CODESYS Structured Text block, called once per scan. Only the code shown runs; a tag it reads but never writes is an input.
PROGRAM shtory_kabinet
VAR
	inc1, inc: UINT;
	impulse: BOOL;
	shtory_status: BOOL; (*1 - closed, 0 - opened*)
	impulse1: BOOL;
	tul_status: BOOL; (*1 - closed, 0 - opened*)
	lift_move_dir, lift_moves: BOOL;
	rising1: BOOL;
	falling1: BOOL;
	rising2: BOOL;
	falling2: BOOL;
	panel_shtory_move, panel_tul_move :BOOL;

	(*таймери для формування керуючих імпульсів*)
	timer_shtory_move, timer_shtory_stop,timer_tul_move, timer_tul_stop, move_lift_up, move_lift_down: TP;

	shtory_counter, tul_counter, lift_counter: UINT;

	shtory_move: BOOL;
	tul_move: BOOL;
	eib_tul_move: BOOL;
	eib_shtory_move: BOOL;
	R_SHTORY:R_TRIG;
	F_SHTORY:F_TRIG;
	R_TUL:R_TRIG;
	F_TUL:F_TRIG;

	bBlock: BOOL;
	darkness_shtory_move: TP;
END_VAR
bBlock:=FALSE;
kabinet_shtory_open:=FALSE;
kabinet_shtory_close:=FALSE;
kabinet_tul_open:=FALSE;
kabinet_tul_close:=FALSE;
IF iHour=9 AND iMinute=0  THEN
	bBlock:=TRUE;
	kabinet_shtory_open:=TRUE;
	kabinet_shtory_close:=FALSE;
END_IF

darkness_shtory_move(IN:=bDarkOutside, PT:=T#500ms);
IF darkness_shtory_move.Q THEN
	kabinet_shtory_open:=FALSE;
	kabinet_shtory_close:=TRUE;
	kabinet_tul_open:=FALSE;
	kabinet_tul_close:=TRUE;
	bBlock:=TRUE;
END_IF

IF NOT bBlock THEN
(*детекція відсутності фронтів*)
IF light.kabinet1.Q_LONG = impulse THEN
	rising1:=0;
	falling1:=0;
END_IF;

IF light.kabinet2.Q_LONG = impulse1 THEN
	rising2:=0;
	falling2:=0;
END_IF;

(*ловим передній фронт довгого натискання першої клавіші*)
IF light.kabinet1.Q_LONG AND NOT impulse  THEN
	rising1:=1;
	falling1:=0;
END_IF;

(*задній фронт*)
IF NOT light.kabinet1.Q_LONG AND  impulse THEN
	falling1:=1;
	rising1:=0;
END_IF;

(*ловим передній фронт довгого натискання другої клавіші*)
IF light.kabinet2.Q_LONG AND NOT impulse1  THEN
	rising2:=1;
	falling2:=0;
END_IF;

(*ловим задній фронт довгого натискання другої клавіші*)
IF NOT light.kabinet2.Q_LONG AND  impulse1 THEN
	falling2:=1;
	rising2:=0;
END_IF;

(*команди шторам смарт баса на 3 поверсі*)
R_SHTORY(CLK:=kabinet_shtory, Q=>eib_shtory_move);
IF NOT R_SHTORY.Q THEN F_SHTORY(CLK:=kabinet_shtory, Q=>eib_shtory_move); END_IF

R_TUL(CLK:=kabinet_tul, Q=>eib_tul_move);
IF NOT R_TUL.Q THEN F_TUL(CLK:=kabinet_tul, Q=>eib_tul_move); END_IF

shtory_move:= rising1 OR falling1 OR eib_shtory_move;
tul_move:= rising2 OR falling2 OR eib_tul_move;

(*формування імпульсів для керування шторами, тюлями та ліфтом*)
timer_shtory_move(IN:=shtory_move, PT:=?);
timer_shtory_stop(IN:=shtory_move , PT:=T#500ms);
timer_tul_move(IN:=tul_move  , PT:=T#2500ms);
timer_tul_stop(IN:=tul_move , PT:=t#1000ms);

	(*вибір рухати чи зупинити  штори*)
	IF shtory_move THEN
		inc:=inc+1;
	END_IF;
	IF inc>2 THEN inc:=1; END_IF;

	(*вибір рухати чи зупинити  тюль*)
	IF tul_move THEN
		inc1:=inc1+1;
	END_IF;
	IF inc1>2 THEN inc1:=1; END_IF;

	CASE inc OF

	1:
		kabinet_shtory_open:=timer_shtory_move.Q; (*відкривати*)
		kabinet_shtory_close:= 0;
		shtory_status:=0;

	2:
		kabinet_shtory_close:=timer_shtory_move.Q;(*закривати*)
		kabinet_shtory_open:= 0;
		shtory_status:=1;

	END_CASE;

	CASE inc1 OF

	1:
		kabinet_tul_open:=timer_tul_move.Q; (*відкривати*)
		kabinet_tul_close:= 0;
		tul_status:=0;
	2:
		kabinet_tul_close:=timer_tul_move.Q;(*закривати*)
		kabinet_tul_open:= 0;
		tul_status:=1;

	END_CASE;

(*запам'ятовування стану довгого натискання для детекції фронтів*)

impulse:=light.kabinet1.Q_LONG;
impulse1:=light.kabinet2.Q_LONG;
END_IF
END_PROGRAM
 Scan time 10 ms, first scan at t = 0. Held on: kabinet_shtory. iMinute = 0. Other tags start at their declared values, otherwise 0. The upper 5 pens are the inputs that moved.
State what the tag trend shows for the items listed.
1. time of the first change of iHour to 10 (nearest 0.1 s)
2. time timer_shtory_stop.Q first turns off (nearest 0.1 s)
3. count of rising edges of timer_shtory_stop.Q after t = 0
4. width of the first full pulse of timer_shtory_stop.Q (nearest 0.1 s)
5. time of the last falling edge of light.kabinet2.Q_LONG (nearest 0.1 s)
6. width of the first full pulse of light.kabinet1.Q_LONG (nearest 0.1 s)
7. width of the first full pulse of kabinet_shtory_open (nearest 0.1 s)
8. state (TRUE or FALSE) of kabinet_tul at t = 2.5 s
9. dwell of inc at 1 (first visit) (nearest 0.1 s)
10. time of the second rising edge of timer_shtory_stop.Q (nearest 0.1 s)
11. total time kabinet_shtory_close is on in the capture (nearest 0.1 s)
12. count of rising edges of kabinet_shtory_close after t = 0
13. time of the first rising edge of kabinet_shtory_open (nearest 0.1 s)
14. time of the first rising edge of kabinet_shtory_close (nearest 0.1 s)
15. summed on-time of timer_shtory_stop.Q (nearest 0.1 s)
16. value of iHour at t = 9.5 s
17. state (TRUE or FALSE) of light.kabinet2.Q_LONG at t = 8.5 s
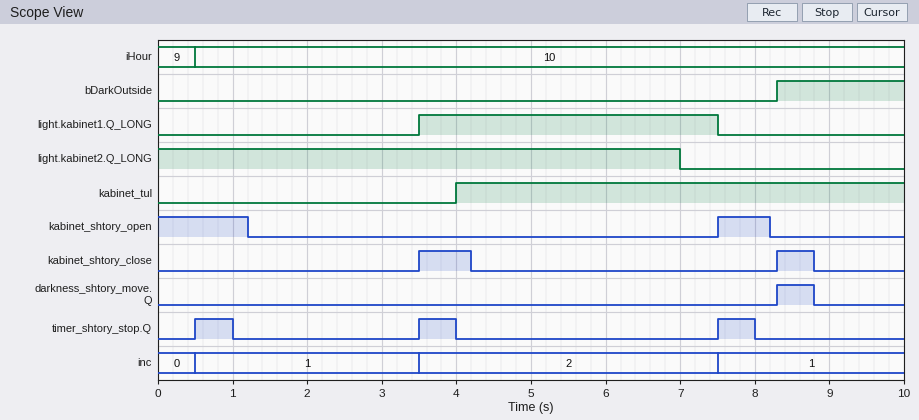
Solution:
0.5 s
1.0 s
3
0.5 s
7.0 s
4.0 s
0.7 s
FALSE
3.0 s
3.5 s
1.2 s
2
7.5 s
3.5 s
1.5 s
10
FALSE
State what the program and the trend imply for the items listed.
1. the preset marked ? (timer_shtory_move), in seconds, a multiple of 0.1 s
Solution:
0.7 s
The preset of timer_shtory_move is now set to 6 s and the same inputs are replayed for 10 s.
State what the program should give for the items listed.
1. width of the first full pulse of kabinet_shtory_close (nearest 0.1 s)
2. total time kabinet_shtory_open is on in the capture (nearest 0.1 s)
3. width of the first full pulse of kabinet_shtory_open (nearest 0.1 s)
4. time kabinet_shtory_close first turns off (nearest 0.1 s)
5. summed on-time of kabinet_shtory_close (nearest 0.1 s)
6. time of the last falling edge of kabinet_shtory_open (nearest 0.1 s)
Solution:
3.0 s
5.5 s
0.8 s
6.5 s
3.5 s
8.3 s
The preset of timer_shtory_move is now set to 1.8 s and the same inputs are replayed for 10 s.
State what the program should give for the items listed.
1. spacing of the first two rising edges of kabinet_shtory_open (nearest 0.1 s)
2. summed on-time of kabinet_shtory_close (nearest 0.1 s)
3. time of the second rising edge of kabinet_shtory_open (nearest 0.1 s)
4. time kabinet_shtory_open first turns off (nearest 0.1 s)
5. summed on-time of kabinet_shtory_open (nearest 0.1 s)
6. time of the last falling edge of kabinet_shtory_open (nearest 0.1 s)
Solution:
1.3 s
2.3 s
8.8 s
2.3 s
3.6 s
9.3 s
